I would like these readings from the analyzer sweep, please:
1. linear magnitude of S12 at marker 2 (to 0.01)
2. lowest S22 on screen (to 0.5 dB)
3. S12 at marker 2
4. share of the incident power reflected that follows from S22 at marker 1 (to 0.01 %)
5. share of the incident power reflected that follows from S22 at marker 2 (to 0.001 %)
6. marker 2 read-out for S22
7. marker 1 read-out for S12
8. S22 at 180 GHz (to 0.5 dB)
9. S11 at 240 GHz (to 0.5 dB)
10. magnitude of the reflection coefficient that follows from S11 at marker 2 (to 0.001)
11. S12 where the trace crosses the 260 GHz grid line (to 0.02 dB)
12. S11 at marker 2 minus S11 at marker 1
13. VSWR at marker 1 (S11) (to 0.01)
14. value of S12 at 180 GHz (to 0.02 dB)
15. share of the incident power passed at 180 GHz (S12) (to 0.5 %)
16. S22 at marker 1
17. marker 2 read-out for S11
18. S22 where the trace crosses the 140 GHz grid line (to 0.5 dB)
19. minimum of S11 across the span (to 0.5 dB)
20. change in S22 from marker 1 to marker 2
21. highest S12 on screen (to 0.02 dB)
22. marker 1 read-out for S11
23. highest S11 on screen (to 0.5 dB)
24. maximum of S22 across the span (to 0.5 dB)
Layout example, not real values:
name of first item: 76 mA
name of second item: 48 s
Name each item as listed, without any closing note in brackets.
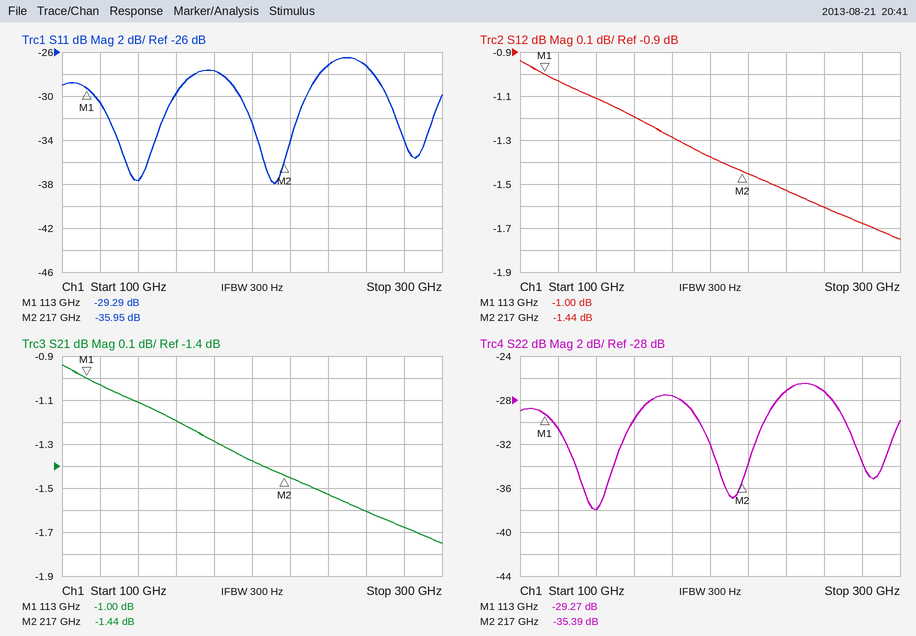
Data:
linear magnitude of S12 at marker 2: 0.85
lowest S22 on screen: -38.0 dB
S12 at marker 2: -1.44 dB
share of the incident power reflected that follows from S22 at marker 1: 0.12 %
share of the incident power reflected that follows from S22 at marker 2: 0.029 %
marker 2 read-out for S22: -35.39 dB
marker 1 read-out for S12: -1.00 dB
S22 at 180 GHz: -27.5 dB
S11 at 240 GHz: -27.0 dB
magnitude of the reflection coefficient that follows from S11 at marker 2: 0.016
S12 where the trace crosses the 260 GHz grid line: -1.60 dB
S11 at marker 2 minus S11 at marker 1: -6.66 dB
VSWR at marker 1 (S11): 1.07
value of S12 at 180 GHz: -1.28 dB
share of the incident power passed at 180 GHz (S12): 74.5 %
S22 at marker 1: -29.27 dB
marker 2 read-out for S11: -35.95 dB
S22 where the trace crosses the 140 GHz grid line: -38.0 dB
minimum of S11 across the span: -38.0 dB
change in S22 from marker 1 to marker 2: -6.12 dB
highest S12 on screen: -0.94 dB
marker 1 read-out for S11: -29.29 dB
highest S11 on screen: -26.5 dB
maximum of S22 across the span: -26.5 dB
